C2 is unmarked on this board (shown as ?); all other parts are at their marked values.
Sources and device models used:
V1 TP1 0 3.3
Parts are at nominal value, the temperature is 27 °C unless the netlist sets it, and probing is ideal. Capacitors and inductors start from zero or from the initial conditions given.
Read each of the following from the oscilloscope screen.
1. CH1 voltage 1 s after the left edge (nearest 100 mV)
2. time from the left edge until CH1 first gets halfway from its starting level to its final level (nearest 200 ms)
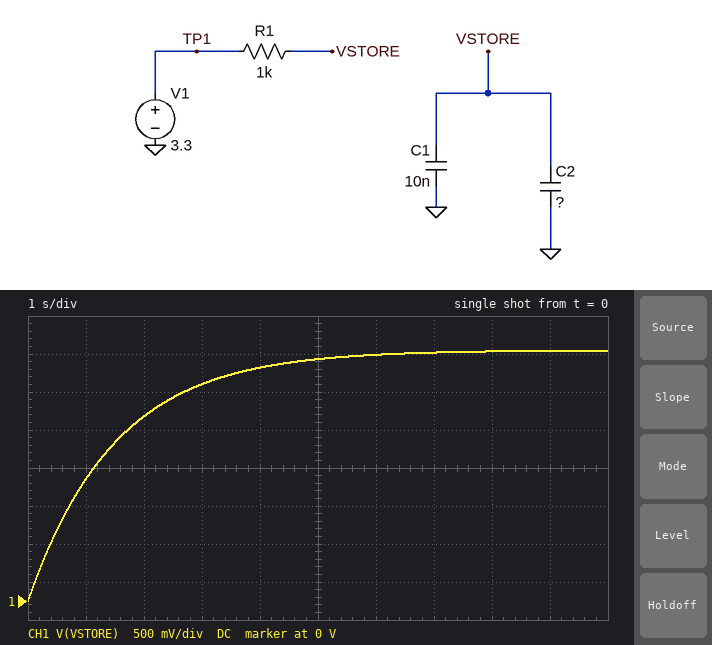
1.6 V
1.0 s
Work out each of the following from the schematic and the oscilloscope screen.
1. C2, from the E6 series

1.5 mF
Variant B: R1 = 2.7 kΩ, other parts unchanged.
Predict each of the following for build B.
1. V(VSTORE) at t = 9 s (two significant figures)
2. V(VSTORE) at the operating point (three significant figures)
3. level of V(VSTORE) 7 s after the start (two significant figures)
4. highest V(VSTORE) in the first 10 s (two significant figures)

2.9 V
3.30 V
2.7 V
3.0 V
